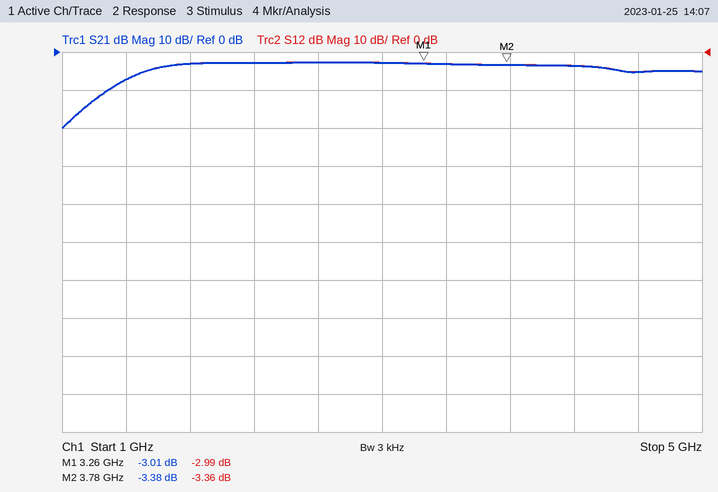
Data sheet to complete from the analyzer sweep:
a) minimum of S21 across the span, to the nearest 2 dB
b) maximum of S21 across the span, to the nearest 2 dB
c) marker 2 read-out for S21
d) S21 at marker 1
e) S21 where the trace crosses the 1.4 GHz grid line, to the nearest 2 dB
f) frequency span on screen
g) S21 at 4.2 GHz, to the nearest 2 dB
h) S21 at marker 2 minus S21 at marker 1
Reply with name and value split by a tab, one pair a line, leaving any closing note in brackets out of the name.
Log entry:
minimum of S21 across the span, to the nearest 2 dB	-20 dB
maximum of S21 across the span, to the nearest 2 dB	-2 dB
marker 2 read-out for S21	-3.38 dB
S21 at marker 1	-3.01 dB
S21 where the trace crosses the 1.4 GHz grid line, to the nearest 2 dB	-8 dB
frequency span on screen	4 GHz
S21 at 4.2 GHz, to the nearest 2 dB	-4 dB
S21 at marker 2 minus S21 at marker 1	-0.37 dB
